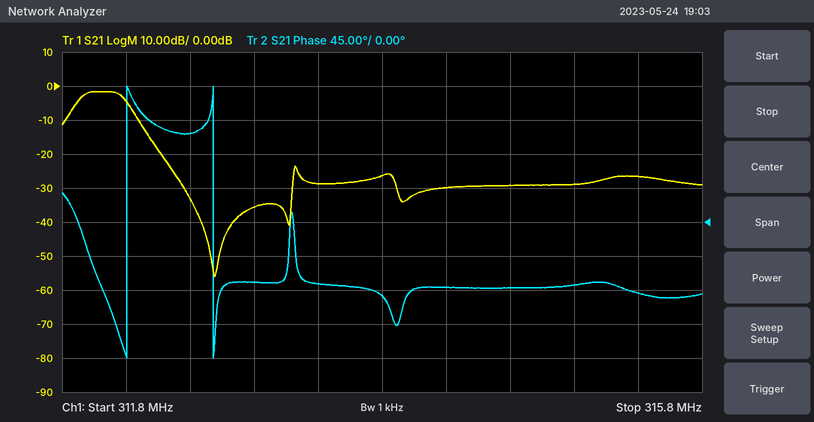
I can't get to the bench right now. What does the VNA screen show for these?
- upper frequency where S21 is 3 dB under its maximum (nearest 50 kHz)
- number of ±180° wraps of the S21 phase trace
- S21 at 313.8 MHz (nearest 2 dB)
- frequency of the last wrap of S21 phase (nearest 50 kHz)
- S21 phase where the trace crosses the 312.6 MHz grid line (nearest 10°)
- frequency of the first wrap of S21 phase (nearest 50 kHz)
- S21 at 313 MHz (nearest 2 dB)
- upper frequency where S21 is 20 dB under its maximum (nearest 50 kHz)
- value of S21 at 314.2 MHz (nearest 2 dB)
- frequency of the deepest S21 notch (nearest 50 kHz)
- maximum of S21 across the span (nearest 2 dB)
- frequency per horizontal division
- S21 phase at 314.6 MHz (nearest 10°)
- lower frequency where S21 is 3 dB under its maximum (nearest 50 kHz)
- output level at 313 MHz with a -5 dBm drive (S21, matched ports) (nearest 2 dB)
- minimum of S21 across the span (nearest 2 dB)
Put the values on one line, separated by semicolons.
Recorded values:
312.20 MHz; 2; -26 dB; 312.75 MHz; 120°; 312.20 MHz; -36 dB; 312.45 MHz; -30 dB; 312.75 MHz; -2 dB; 400 kHz; -90°; 311.90 MHz; -40 dBm; -56 dB
